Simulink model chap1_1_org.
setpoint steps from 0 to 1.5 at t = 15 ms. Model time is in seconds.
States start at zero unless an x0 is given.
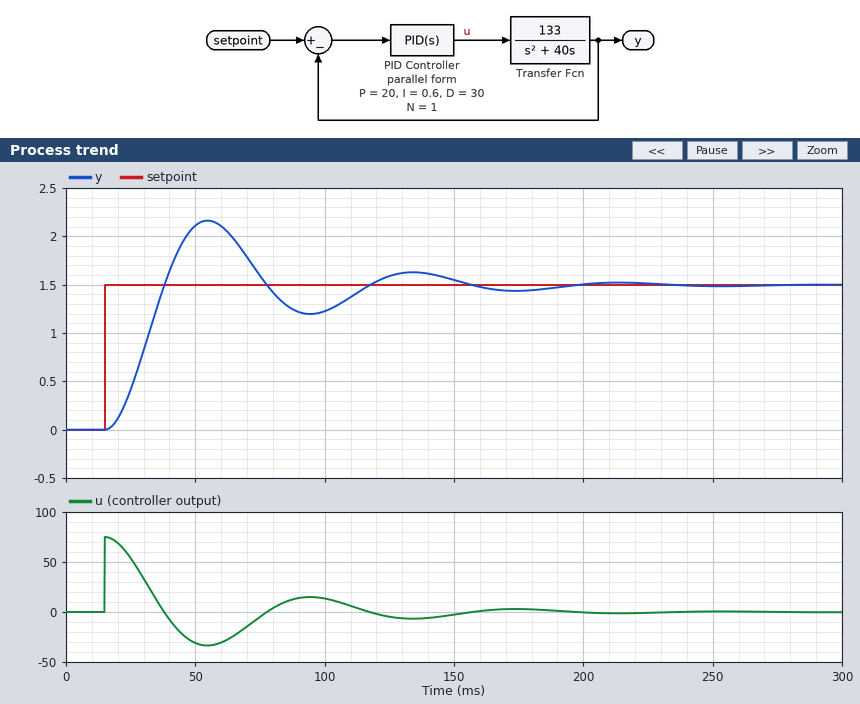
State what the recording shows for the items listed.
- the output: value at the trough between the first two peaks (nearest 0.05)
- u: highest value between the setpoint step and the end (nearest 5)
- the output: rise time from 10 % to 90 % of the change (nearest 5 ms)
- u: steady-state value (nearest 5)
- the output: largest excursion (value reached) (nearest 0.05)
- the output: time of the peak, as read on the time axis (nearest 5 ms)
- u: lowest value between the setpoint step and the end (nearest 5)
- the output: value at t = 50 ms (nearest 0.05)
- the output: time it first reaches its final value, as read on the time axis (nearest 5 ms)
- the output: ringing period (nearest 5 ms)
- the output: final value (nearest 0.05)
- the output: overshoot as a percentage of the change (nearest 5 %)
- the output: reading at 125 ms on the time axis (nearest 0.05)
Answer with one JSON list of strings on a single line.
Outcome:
["1.20", "75", "15 ms", "0", "2.15", "55 ms", "-35", "2.10", "40 ms", "80 ms", "1.50", "45 %", "1.60"]
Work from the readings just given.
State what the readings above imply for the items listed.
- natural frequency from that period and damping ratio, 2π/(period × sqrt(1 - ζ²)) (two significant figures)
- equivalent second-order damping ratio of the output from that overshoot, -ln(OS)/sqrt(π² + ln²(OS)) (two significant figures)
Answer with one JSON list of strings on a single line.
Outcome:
["0.081 rad/ms", "0.25"]
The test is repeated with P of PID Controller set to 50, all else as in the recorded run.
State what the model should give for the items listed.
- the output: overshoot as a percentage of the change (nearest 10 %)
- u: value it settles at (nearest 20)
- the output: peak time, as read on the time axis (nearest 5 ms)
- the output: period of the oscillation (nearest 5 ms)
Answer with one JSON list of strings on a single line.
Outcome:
["50 %", "0", "45 ms", "60 ms"]
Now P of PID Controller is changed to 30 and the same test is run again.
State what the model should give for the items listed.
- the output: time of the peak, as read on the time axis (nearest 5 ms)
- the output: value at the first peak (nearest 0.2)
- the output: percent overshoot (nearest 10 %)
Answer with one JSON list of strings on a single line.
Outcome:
["50 ms", "2.2", "50 %"]
